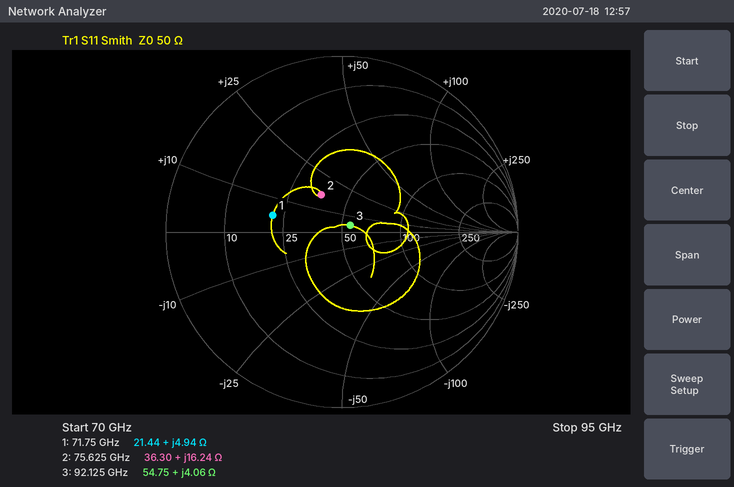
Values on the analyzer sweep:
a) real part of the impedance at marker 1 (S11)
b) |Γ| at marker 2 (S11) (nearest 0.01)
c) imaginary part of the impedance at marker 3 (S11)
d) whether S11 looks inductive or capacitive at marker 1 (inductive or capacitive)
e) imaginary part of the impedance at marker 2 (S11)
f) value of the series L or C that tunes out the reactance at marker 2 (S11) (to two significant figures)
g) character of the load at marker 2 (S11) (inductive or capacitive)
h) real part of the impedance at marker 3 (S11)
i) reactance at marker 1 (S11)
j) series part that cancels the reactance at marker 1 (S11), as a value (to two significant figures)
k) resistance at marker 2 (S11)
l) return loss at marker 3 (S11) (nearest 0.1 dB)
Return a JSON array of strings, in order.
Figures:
["21.44 Ω", "0.24", "+4.06 Ω", "inductive", "+16.24 Ω", "130 fF", "inductive", "54.75 Ω", "+4.94 Ω", "450 fF", "36.30 Ω", "24.5 dB"]
